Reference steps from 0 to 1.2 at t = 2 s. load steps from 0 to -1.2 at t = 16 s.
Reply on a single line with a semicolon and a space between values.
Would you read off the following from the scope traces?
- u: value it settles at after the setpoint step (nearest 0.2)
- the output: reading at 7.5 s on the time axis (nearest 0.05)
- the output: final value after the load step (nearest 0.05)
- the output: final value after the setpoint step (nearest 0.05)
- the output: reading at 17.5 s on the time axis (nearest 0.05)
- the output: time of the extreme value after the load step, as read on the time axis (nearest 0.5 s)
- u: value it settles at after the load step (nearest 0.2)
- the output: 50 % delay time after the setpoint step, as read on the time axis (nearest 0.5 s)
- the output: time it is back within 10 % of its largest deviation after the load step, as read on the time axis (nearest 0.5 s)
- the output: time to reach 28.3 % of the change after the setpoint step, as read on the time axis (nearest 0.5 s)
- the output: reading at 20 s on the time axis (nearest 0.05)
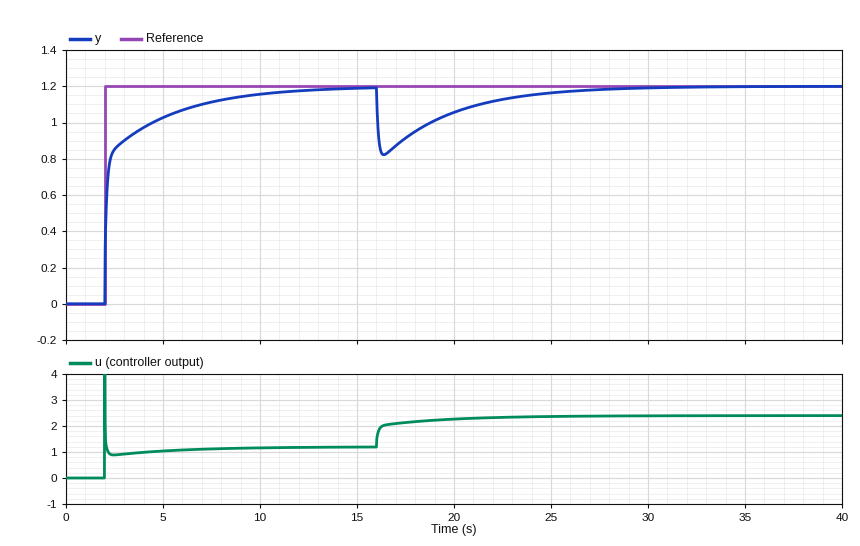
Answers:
1.2; 1.10; 1.20; 1.20; 0.90; 16.5 s; 2.4; 2.0 s; 25.0 s; 2.0 s; 1.05
